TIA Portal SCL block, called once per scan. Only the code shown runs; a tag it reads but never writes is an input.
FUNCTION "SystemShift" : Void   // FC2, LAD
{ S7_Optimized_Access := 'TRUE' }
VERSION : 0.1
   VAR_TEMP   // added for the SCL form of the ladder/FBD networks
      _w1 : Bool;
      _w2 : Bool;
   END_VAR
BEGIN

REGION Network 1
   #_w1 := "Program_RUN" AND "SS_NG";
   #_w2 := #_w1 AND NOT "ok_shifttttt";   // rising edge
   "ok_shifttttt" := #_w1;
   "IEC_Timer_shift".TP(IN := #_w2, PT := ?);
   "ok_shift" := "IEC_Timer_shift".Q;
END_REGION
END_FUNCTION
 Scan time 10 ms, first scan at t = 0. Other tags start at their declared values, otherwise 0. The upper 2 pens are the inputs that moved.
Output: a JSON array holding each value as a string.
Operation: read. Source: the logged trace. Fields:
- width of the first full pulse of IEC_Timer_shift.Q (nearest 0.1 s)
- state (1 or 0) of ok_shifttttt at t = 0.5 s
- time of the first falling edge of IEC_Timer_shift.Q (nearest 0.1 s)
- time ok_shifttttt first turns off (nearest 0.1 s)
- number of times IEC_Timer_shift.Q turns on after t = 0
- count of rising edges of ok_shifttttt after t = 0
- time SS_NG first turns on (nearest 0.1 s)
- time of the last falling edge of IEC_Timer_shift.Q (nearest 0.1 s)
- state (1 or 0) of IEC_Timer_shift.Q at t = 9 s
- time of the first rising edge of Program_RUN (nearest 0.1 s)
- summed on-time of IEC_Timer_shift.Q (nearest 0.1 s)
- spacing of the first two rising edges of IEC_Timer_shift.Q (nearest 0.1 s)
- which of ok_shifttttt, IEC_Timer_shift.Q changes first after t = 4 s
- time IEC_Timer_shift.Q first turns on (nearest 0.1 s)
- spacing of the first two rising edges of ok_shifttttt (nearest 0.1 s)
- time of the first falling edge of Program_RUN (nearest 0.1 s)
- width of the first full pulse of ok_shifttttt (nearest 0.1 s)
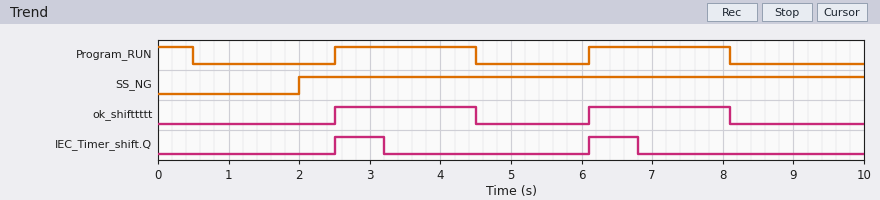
["0.7 s", "0", "3.2 s", "4.5 s", "2", "2", "2.0 s", "6.8 s", "0", "2.5 s", "1.4 s", "3.6 s", "ok_shifttttt", "2.5 s", "3.6 s", "0.5 s", "2.0 s"]
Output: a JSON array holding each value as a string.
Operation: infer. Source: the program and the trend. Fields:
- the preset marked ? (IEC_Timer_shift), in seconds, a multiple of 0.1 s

["0.7 s"]
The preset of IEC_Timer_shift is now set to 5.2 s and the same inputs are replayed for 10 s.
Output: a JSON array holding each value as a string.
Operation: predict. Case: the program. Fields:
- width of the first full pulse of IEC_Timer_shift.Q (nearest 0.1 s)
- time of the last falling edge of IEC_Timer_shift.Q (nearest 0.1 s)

["5.2 s", "7.7 s"]
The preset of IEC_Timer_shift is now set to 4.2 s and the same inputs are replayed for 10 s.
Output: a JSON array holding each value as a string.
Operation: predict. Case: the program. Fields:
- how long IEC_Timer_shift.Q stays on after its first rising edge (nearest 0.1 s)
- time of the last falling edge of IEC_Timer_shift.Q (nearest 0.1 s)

["4.2 s", "6.7 s"]
